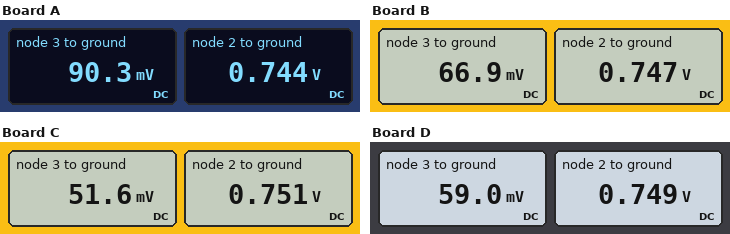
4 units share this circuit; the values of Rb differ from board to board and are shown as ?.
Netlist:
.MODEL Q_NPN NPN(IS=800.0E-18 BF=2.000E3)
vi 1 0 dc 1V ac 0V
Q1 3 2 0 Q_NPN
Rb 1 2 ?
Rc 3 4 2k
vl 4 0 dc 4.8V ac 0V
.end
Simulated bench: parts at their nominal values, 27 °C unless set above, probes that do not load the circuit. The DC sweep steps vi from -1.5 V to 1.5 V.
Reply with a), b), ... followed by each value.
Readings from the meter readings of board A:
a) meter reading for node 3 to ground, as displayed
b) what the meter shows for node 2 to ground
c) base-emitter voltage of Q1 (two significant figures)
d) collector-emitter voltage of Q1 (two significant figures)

a) 90.3 mV
b) 0.744 V
c) 740 mV
d) 90 mV
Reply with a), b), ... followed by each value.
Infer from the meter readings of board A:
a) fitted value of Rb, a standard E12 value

a) 3.3 kΩ
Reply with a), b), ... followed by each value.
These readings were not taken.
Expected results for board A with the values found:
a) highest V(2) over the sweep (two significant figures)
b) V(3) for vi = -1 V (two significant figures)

a) 750 mV
b) 4.8 V
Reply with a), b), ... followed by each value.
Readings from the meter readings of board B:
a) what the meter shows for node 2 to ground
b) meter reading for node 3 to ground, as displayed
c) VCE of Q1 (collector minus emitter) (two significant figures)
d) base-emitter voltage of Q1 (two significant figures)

a) 0.747 V
b) 66.9 mV
c) 67 mV
d) 750 mV
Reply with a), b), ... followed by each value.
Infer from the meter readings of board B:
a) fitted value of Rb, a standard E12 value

a) 1.2 kΩ
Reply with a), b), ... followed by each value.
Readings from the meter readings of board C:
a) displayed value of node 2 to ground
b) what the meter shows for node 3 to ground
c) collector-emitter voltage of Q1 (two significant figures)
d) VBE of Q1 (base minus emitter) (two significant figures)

a) 0.751 V
b) 51.6 mV
c) 52 mV
d) 750 mV
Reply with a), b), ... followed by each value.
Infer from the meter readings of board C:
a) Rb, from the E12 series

a) 560 Ω
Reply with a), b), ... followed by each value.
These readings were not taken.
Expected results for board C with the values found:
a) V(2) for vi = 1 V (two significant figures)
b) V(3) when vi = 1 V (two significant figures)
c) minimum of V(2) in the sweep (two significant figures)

a) 750 mV
b) 52 mV
c) -1.5 V
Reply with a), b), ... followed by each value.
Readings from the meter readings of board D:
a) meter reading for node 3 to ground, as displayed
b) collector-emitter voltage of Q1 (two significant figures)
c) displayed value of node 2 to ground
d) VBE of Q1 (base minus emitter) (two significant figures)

a) 59.0 mV
b) 59 mV
c) 0.749 V
d) 750 mV
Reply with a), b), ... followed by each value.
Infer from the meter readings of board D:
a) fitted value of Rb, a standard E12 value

a) 820 Ω
